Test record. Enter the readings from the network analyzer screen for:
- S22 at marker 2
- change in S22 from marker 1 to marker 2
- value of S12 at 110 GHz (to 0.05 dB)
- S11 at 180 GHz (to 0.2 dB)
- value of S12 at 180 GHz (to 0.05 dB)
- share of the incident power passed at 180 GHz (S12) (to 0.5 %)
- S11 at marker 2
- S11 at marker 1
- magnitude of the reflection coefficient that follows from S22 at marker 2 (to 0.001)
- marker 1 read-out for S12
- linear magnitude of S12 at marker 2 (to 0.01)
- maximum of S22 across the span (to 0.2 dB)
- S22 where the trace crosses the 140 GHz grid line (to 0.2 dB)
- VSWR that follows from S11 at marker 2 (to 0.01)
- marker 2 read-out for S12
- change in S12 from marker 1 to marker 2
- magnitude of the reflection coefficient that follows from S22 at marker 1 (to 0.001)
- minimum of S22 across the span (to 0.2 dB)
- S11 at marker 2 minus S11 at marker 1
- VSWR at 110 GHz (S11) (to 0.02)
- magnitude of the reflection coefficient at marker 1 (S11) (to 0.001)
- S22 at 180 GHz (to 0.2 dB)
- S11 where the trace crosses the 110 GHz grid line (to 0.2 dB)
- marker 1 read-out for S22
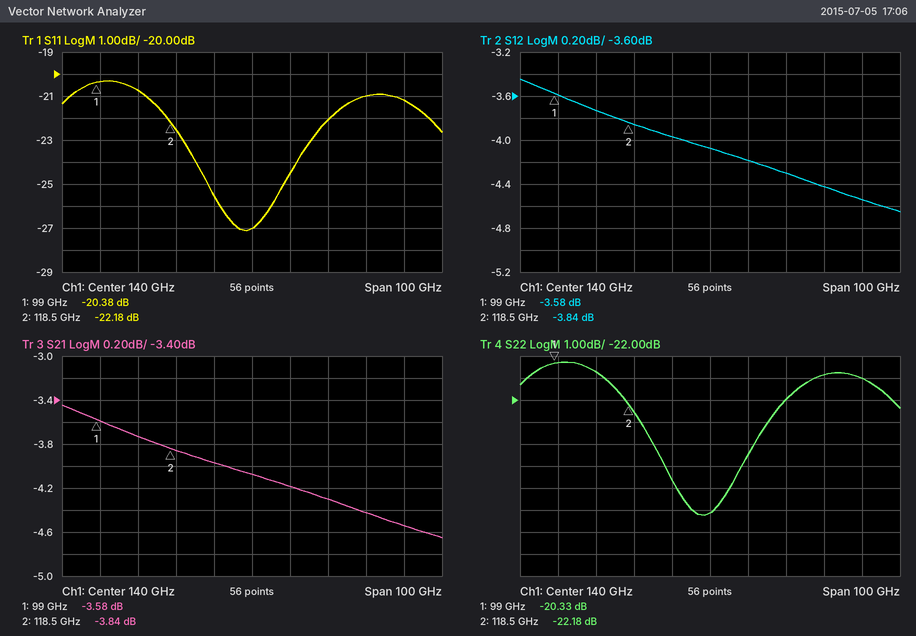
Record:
-22.18 dB
-1.85 dB
-3.75 dB
-21.2 dB
-4.55 dB
35.0 %
-22.18 dB
-20.38 dB
0.078
-3.58 dB
0.64
-20.2 dB
-27.2 dB
1.17
-3.84 dB
-0.26 dB
0.096
-27.2 dB
-1.80 dB
1.20
0.096
-21.0 dB
-20.8 dB
-20.33 dB
